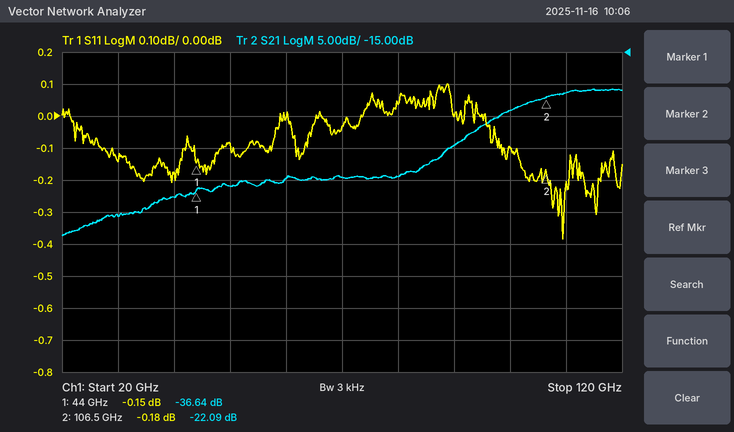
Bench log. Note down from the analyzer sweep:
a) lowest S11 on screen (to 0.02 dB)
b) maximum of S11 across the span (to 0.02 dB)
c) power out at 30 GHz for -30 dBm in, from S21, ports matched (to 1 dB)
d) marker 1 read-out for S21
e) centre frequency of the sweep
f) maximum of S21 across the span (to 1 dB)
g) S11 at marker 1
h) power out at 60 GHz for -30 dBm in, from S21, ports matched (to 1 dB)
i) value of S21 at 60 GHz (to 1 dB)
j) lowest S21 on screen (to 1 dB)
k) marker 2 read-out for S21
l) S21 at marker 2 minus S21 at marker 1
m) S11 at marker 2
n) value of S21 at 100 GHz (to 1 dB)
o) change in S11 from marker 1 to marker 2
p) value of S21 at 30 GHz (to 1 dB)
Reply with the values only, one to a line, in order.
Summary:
-0.38 dB
0.10 dB
-71 dBm
-36.64 dB
70 GHz
-21 dB
-0.15 dB
-65 dBm
-35 dB
-44 dB
-22.09 dB
14.55 dB
-0.18 dB
-24 dB
-0.03 dB
-41 dB
